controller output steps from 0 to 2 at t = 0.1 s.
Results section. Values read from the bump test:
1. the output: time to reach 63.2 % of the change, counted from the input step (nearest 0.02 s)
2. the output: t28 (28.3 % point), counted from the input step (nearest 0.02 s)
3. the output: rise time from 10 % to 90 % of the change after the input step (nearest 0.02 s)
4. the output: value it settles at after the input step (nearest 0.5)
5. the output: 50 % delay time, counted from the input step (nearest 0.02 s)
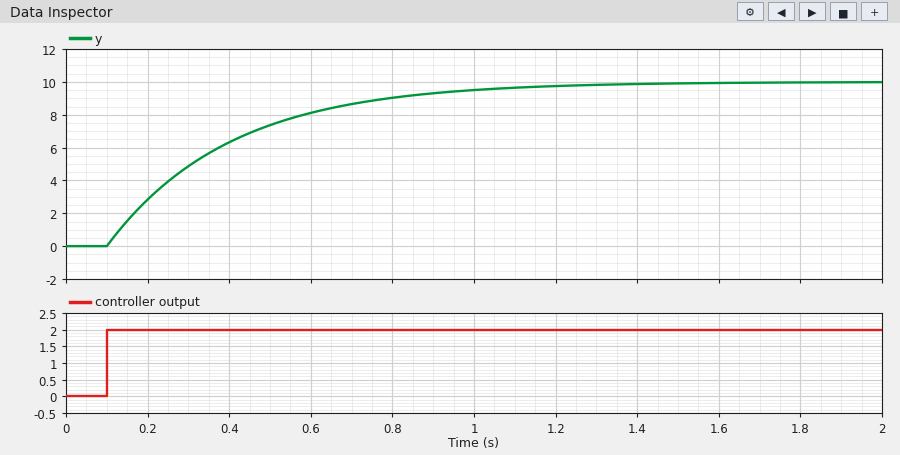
0.30 s
0.10 s
0.66 s
10.0
0.20 s
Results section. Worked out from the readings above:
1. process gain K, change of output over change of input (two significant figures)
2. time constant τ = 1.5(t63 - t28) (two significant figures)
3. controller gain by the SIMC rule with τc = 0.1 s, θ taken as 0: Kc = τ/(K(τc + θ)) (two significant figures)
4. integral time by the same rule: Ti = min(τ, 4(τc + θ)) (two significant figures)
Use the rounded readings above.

5.0
0.30 s
0.60
0.30 s
